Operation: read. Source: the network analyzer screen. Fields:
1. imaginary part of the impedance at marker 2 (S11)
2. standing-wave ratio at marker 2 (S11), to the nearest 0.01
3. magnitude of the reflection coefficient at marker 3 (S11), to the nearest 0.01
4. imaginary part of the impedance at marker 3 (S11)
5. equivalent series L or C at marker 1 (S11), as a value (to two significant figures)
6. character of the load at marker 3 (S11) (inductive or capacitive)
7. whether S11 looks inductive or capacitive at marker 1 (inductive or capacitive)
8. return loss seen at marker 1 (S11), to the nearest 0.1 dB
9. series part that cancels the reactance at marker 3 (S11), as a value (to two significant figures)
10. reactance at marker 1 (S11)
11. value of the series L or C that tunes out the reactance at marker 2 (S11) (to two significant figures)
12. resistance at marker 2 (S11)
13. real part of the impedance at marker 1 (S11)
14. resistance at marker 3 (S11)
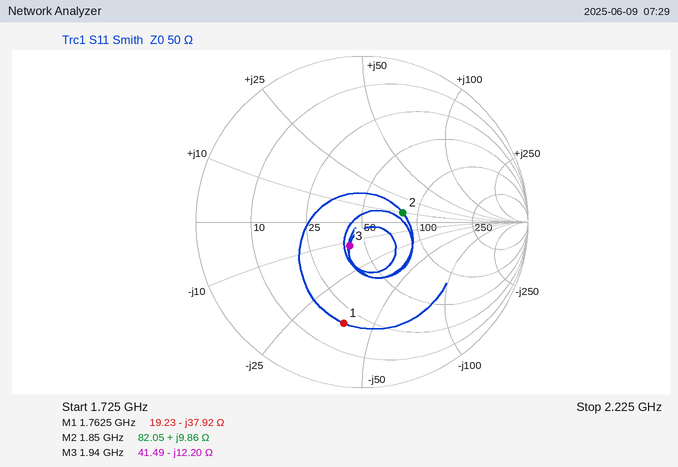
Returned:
+9.86 Ω
1.68
0.16
-12.20 Ω
2.4 pF
capacitive
capacitive
4.2 dB
1.0 nH
-37.92 Ω
8.7 pF
82.05 Ω
19.23 Ω
41.49 Ω
